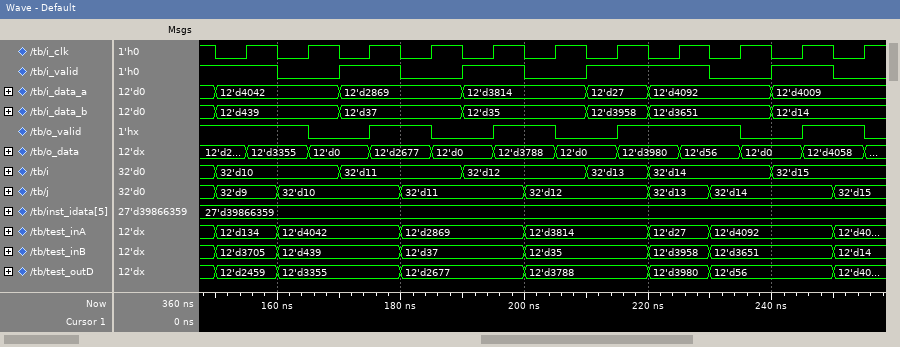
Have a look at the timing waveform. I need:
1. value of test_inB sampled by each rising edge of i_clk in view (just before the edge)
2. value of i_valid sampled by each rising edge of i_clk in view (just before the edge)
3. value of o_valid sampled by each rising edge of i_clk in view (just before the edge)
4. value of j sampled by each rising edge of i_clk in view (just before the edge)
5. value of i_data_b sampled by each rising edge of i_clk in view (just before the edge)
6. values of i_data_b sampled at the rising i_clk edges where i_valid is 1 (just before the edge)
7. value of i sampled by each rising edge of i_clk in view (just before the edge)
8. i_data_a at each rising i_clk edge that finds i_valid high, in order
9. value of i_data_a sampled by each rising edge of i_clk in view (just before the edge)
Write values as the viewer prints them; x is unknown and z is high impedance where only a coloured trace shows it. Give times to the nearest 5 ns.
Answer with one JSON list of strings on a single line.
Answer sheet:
["12'd3705, 12'd439, 12'd439, 12'd37, 12'd37, 12'd35, 12'd35, 12'd3958, 12'd3651, 12'd3651, 12'd14", "1 0 1 0 1 0 1 1 0 1 0", "1 1 0 1 0 1 0 1 1 0 1", "32'd9, 32'd10, 32'd10, 32'd11, 32'd11, 32'd12, 32'd12, 32'd13, 32'd14, 32'd14, 32'd15", "12'd439, 12'd439, 12'd37, 12'd37, 12'd35, 12'd35, 12'd3958, 12'd3651, 12'd3651, 12'd14, 12'd14", "12'd439, 12'd37, 12'd35, 12'd3958, 12'd3651, 12'd14", "32'd10, 32'd10, 32'd11, 32'd11, 32'd12, 32'd12, 32'd13, 32'd14, 32'd14, 32'd15, 32'd15", "12'd4042, 12'd2869, 12'd3814, 12'd27, 12'd4092, 12'd4009", "12'd4042, 12'd4042, 12'd2869, 12'd2869, 12'd3814, 12'd3814, 12'd27, 12'd4092, 12'd4092, 12'd4009, 12'd4009"]
